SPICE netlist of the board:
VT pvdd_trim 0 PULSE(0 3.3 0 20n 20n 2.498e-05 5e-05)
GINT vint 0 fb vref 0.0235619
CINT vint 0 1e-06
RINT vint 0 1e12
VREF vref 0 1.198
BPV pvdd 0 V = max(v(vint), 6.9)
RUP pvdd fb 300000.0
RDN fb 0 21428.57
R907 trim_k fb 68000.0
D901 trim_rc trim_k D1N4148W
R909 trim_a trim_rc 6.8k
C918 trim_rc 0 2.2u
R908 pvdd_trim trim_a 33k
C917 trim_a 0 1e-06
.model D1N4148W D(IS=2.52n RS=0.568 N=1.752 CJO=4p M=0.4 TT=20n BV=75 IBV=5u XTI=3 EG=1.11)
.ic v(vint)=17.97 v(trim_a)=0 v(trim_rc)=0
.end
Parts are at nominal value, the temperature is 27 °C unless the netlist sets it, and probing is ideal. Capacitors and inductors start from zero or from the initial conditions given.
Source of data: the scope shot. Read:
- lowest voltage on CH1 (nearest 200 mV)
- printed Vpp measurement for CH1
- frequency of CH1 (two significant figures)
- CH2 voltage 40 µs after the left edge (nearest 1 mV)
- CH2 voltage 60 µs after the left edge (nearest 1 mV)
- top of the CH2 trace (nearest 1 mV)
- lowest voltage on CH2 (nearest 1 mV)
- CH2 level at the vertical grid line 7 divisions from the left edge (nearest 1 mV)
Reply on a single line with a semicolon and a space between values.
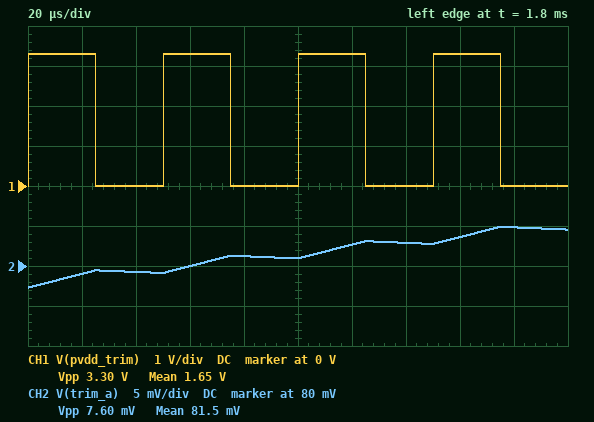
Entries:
0 V; 3.30 V; 20 kHz; 79 mV; 80 mV; 85 mV; 77 mV; 83 mV
